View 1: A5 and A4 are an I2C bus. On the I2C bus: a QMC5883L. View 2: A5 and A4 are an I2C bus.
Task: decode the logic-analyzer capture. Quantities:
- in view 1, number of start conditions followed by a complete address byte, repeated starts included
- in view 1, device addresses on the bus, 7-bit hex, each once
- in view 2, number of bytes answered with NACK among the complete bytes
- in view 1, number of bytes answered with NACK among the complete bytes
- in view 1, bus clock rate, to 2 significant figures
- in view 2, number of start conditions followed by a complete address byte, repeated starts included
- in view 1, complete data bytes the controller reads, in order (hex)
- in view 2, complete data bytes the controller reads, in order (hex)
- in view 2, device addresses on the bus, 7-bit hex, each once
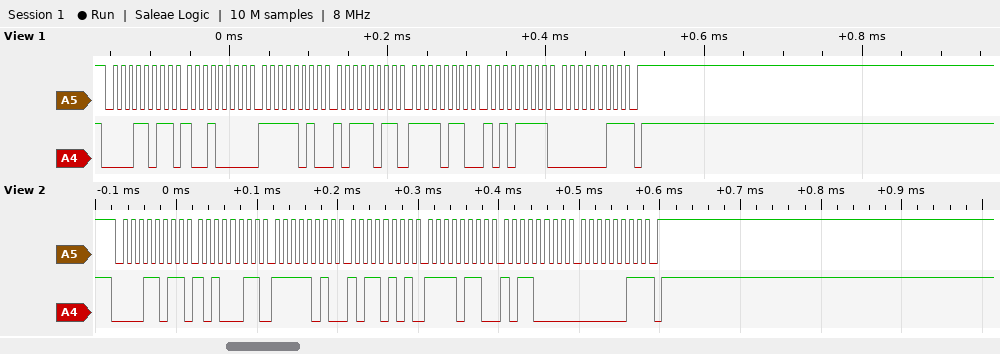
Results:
1
0x0D
1
1
100 kHz
1
90 FA BB F6 AF 03
A3 FA B5 F6 B0 03
0x0D
